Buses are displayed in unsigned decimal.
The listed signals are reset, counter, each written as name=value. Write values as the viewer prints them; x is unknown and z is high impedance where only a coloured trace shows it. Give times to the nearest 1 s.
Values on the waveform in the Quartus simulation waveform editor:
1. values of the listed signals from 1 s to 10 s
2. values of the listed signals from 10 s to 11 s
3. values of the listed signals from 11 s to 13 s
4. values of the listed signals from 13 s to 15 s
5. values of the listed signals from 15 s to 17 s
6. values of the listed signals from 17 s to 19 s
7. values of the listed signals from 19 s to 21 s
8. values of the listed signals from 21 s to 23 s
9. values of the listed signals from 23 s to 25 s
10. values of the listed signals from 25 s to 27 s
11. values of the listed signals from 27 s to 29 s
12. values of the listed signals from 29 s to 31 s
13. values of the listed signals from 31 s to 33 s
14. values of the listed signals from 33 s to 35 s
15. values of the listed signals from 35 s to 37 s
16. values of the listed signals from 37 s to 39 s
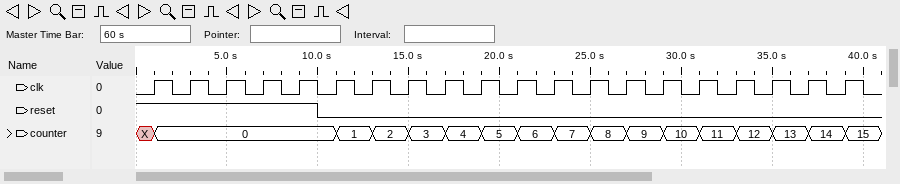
reset=1, counter=0
reset=0, counter=0
reset=0, counter=1
reset=0, counter=2
reset=0, counter=3
reset=0, counter=4
reset=0, counter=5
reset=0, counter=6
reset=0, counter=7
reset=0, counter=8
reset=0, counter=9
reset=0, counter=10
reset=0, counter=11
reset=0, counter=12
reset=0, counter=13
reset=0, counter=14
